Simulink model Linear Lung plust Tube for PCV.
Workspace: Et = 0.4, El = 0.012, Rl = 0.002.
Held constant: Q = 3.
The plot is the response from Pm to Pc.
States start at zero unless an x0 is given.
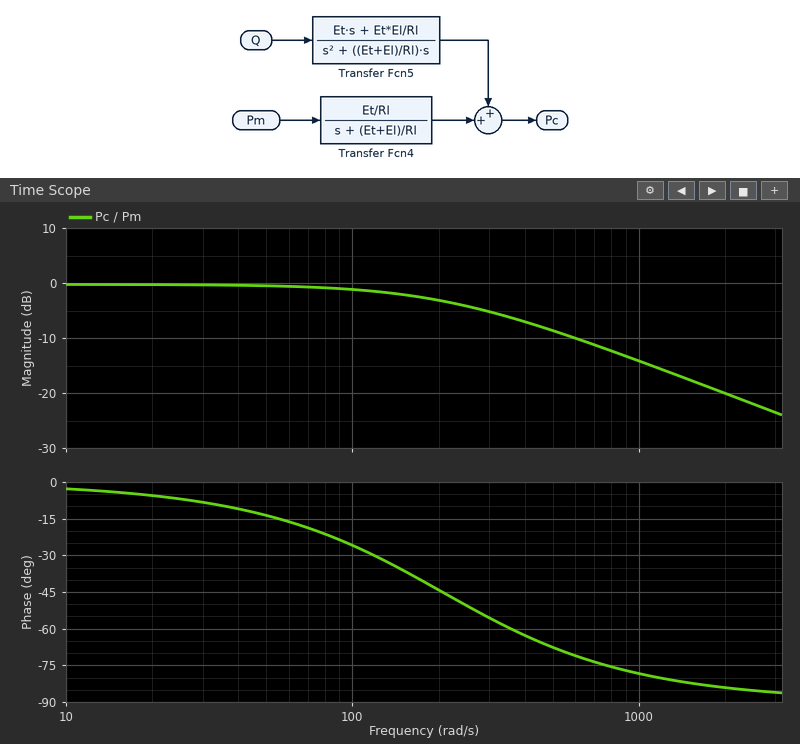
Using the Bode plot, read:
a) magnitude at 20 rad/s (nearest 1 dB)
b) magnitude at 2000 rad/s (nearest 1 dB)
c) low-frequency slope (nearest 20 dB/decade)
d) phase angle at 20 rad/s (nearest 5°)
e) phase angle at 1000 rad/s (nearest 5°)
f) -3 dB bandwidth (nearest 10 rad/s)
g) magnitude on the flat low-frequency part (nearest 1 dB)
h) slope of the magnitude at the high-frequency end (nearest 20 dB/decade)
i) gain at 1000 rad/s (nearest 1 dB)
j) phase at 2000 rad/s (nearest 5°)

0 dB
-20 dB
0 dB/decade
-5°
-80°
210 rad/s
0 dB
-20 dB/decade
-14 dB
-85°
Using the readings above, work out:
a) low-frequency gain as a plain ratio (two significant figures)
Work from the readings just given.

1.0
